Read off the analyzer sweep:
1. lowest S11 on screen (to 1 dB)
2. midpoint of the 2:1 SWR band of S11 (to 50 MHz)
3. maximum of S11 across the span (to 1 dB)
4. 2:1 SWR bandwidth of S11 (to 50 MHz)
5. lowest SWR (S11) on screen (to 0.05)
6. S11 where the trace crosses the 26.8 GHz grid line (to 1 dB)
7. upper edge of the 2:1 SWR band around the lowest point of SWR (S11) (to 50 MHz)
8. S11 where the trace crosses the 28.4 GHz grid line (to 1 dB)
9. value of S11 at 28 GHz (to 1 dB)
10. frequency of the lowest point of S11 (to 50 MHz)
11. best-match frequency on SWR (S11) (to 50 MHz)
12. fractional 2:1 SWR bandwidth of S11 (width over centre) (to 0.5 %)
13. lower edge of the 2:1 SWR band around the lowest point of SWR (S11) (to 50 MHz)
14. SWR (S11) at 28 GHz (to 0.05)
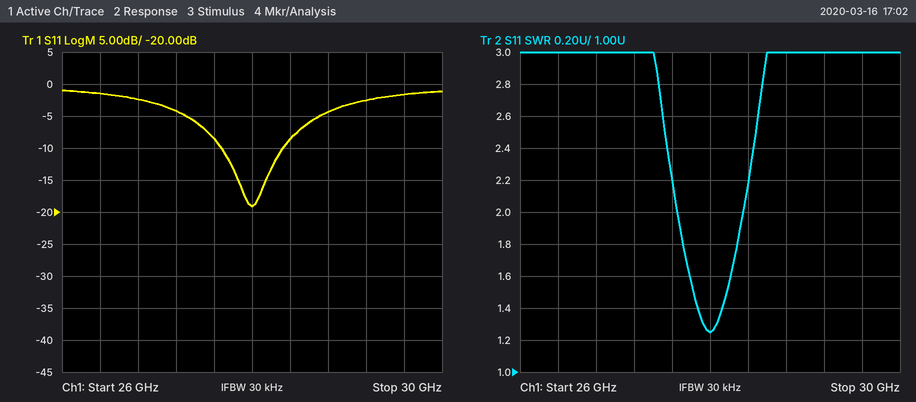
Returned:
-19 dB
28.00 GHz
-1 dB
700 MHz
1.25
-2 dB
28.35 GHz
-9 dB
-19 dB
28.00 GHz
28.00 GHz
2.5 %
27.65 GHz
1.25
